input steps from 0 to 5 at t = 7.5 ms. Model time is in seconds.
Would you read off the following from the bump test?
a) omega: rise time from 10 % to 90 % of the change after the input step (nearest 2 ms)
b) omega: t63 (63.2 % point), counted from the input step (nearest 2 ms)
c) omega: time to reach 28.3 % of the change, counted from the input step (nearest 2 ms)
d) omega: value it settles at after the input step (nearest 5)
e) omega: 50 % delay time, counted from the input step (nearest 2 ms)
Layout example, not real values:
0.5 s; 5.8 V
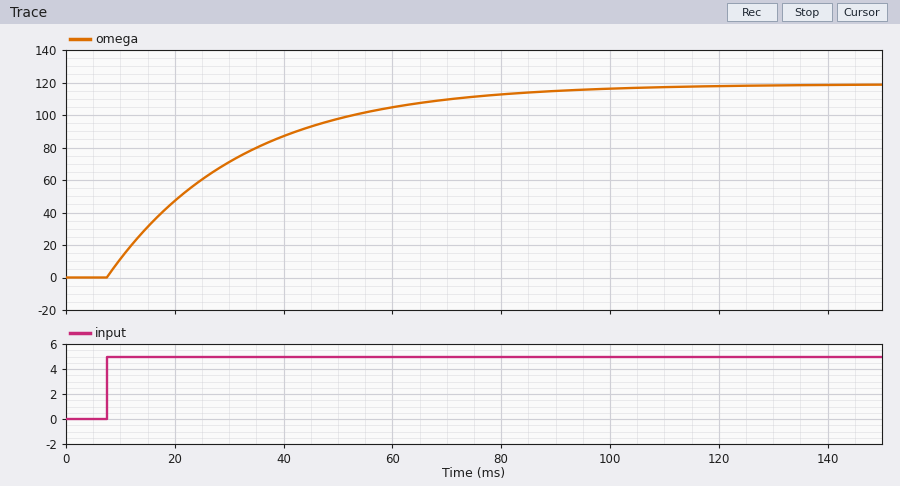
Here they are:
54 ms; 24 ms; 8 ms; 120; 18 ms
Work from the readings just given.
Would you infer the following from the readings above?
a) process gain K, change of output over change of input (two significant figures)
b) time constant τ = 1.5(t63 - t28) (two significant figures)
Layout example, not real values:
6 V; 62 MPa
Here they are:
24; 24 ms
